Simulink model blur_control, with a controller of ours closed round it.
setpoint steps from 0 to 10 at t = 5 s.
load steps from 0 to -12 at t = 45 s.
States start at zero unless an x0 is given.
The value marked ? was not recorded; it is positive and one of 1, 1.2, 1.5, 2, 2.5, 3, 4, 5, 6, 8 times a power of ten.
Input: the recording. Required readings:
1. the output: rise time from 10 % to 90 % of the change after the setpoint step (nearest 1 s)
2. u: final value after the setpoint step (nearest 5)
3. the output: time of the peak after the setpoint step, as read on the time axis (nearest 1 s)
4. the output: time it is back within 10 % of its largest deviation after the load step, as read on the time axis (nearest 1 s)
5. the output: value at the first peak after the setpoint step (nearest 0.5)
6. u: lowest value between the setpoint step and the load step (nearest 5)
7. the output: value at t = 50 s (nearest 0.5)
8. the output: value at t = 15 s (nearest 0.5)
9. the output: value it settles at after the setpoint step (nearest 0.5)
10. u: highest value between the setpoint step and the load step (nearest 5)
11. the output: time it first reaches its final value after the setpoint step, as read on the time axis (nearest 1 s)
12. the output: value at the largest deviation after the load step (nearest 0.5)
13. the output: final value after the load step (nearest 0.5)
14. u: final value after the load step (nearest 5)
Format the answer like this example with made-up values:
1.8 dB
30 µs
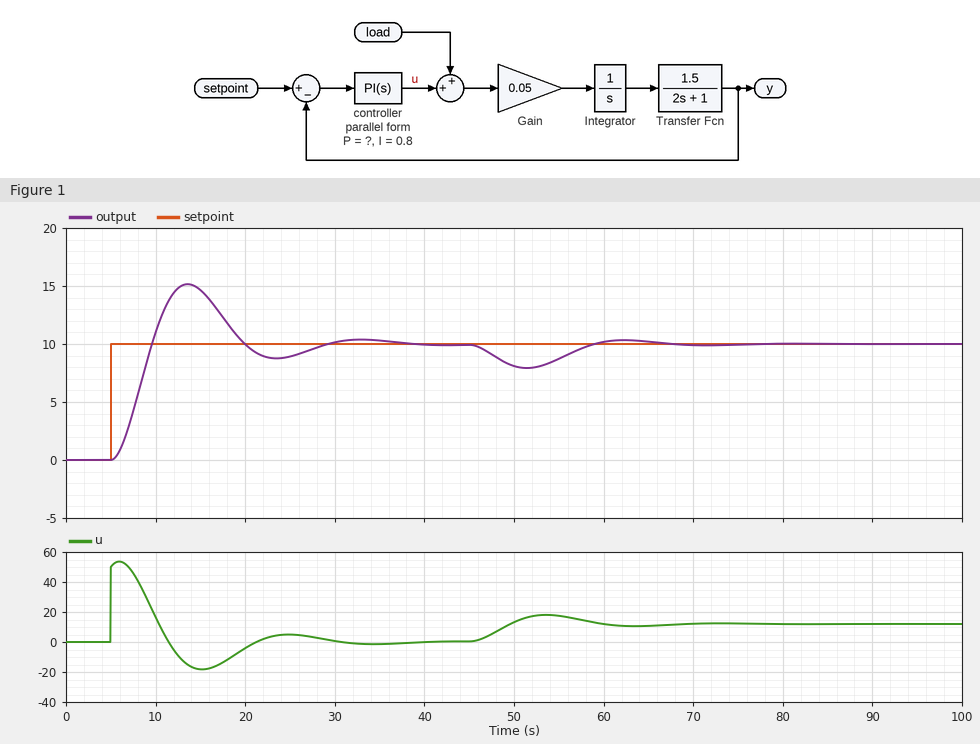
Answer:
3 s
0
14 s
65 s
15.0
-20
8.0
14.5
10.0
55
10 s
8.0
10.0
10
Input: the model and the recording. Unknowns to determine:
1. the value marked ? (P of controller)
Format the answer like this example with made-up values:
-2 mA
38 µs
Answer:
5
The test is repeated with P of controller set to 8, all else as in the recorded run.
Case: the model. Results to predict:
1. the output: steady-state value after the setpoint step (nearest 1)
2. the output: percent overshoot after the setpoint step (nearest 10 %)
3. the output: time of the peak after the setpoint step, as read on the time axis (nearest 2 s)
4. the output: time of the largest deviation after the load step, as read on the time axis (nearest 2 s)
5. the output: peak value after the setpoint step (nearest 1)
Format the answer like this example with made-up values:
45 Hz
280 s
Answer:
10
40 %
12 s
50 s
14
